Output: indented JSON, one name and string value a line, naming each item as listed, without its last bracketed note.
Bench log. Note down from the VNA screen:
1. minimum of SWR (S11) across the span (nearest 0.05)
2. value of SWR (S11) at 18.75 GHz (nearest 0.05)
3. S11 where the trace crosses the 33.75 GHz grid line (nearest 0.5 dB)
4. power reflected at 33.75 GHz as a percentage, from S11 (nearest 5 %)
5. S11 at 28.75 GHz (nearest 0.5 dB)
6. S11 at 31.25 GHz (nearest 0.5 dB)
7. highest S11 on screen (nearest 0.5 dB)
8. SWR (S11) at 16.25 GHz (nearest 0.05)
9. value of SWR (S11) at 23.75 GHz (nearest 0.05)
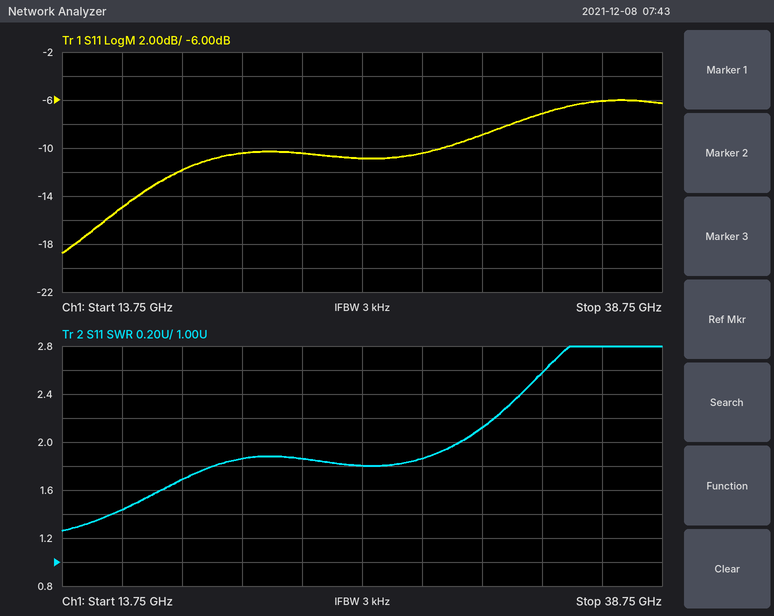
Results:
{
  "minimum of SWR (S11) across the span": "1.25",
  "value of SWR (S11) at 18.75 GHz": "1.70",
  "S11 where the trace crosses the 33.75 GHz grid line": "-7.0 dB",
  "power reflected at 33.75 GHz as a percentage, from S11": "20 %",
  "S11 at 28.75 GHz": "-10.5 dB",
  "S11 at 31.25 GHz": "-9.0 dB",
  "highest S11 on screen": "-6.0 dB",
  "SWR (S11) at 16.25 GHz": "1.45",
  "value of SWR (S11) at 23.75 GHz": "1.85"
}
